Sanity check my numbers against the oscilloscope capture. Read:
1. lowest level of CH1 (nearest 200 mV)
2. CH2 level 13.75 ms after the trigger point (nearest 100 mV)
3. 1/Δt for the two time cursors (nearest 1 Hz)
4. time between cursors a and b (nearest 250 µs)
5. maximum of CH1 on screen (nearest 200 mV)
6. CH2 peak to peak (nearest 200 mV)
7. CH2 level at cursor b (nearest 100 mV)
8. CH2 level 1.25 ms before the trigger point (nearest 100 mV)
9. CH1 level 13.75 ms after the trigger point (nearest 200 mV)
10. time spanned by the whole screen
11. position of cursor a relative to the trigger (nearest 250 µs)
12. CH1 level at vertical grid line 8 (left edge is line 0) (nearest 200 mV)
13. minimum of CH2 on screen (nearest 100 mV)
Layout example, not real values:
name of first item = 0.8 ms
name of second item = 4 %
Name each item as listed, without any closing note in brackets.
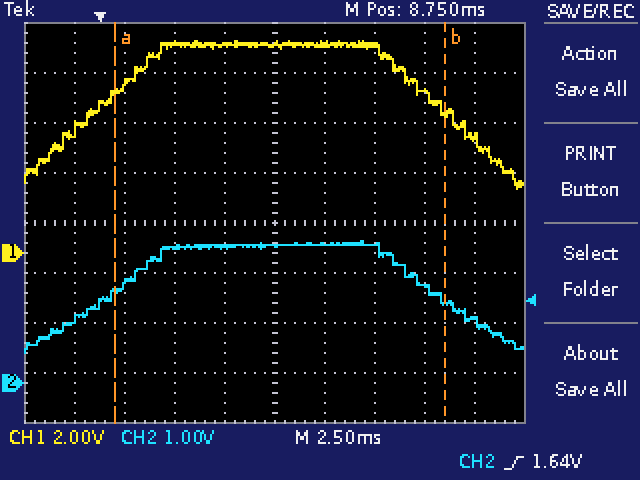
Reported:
lowest level of CH1 = 2.6 V
CH2 level 13.75 ms after the trigger point = 2.8 V
1/Δt for the two time cursors = 61 Hz
time between cursors a and b = 16.50 ms
maximum of CH1 on screen = 8.4 V
CH2 peak to peak = 2.2 V
CH2 level at cursor b = 1.7 V
CH2 level 1.25 ms before the trigger point = 1.3 V
CH1 level 13.75 ms after the trigger point = 8.4 V
time spanned by the whole screen = 25 ms
position of cursor a relative to the trigger = +750 µs
CH1 level at vertical grid line 8 (left edge is line 0) = 6.4 V
minimum of CH2 on screen = 600 mV
